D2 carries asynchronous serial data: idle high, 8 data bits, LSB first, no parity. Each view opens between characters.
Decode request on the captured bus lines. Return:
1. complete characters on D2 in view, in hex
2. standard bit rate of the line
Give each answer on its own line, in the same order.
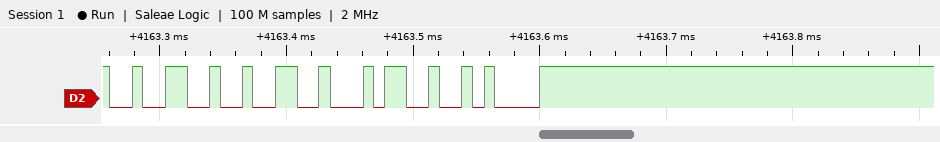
32, 32, 34, 0A
115200 baud
